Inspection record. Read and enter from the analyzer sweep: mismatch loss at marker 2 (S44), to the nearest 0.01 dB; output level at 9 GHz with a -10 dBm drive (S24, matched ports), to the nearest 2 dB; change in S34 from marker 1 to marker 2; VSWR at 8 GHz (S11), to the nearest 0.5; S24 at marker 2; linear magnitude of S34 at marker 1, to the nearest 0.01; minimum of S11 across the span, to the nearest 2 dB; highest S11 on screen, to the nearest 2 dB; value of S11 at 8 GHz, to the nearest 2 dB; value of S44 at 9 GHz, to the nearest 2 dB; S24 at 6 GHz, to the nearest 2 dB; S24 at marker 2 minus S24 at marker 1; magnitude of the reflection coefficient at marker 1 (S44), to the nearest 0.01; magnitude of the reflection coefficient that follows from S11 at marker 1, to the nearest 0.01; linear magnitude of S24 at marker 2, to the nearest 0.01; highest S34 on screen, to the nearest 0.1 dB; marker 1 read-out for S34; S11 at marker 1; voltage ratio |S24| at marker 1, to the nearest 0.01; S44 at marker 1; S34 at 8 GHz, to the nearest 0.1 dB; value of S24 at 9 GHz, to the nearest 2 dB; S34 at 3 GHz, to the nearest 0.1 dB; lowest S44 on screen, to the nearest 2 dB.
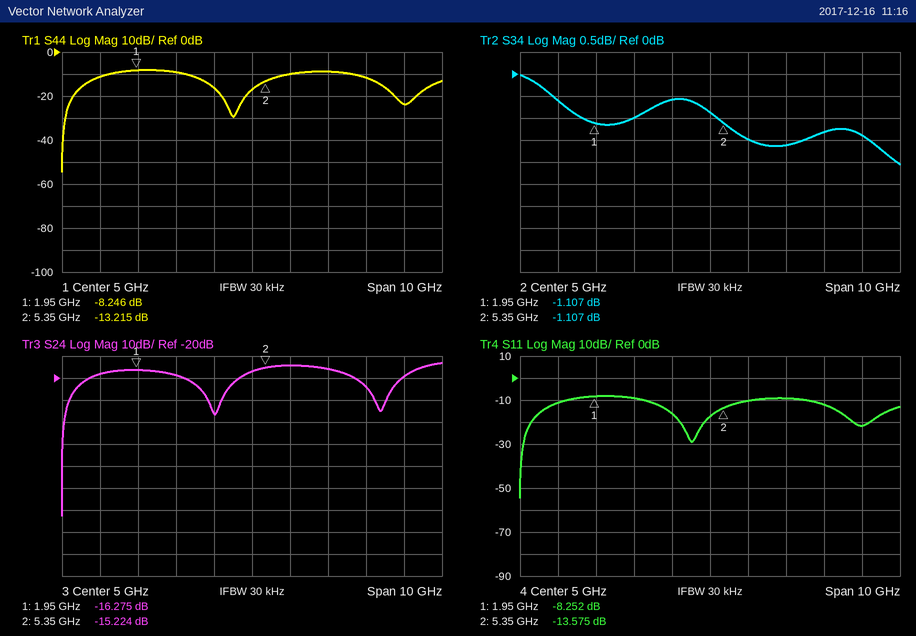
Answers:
0.21 dB
-30 dBm
0.000 dB
1.5
-15.224 dB
0.88
-54 dB
-8 dB
-12 dB
-24 dB
-14 dB
1.051 dB
0.39
0.39
0.17
0.0 dB
-1.107 dB
-8.252 dB
0.15
-8.246 dB
-1.3 dB
-20 dB
-1.0 dB
-54 dB
